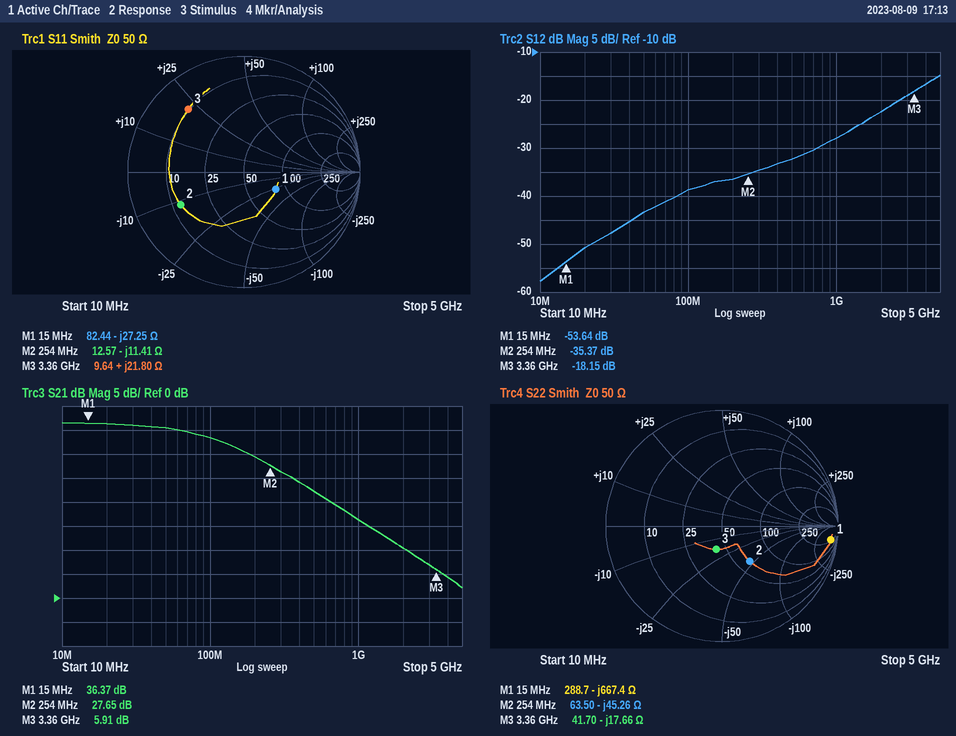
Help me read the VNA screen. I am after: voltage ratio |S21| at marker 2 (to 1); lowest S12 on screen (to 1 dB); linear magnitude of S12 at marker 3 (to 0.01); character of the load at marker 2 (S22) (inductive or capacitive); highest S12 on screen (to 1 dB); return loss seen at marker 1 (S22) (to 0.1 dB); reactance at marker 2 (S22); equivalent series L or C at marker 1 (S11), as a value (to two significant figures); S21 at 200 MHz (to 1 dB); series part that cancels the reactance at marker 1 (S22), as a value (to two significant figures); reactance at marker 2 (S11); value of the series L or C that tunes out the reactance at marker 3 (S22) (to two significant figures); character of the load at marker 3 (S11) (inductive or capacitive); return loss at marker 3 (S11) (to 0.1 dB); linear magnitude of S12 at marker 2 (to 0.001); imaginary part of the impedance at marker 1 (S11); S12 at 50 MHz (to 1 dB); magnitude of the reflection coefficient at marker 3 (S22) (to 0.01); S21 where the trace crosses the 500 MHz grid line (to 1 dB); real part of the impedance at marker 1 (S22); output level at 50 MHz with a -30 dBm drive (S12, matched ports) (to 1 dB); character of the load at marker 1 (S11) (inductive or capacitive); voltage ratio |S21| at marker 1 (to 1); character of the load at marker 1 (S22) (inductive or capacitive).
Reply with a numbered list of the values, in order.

1. 24
2. -58 dB
3. 0.12
4. capacitive
5. -15 dB
6. 0.5 dB
7. -45.26 Ω
8. 390 pF
9. 29 dB
10. 7.1 µH
11. -11.41 Ω
12. 840 pH
13. inductive
14. 2.8 dB
15. 0.017
16. -27.25 Ω
17. -43 dB
18. 0.21
19. 22 dB
20. 288.7 Ω
21. -73 dBm
22. capacitive
23. 66
24. capacitive
